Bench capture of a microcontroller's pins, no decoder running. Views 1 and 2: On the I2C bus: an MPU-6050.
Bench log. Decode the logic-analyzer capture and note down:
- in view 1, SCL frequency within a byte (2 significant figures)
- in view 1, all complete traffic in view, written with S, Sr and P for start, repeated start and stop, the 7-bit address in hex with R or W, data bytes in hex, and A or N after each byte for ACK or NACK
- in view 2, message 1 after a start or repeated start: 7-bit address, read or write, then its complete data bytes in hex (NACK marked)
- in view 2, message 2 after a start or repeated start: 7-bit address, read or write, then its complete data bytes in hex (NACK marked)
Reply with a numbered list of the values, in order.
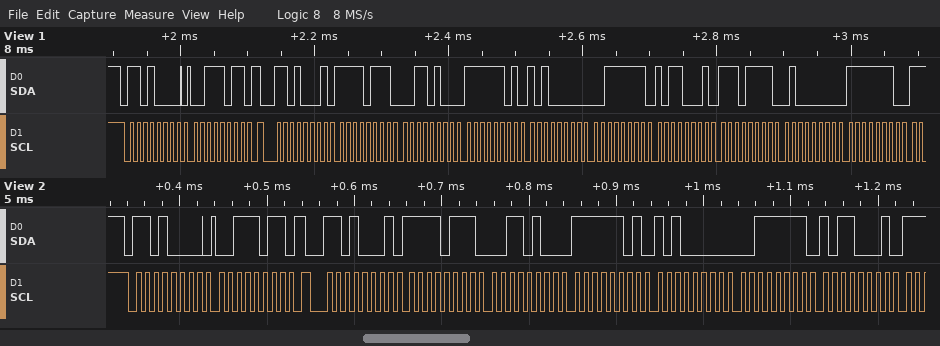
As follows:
1. 100 kHz
2. S 68W A 3B A Sr 68R A F7 A 34 A FD A A0 A 3F A B1 A EF A 40 A FE A
3. 0x68 write: 3B
4. 0x68 read: F7 34 FD A0 3F B1
